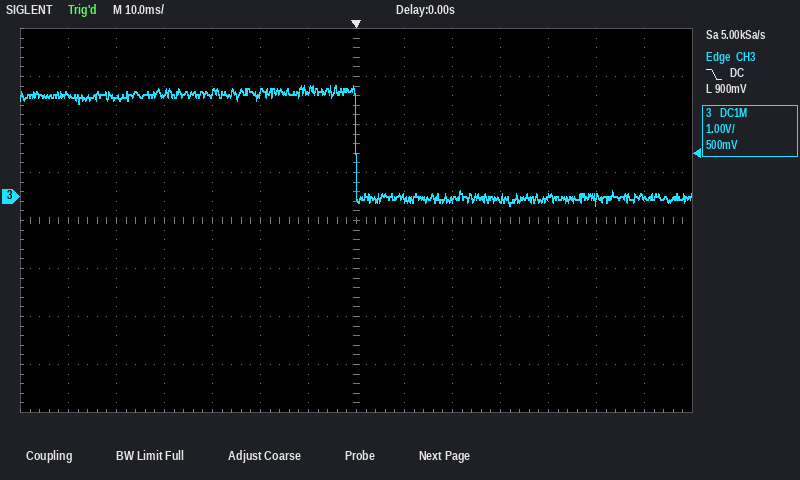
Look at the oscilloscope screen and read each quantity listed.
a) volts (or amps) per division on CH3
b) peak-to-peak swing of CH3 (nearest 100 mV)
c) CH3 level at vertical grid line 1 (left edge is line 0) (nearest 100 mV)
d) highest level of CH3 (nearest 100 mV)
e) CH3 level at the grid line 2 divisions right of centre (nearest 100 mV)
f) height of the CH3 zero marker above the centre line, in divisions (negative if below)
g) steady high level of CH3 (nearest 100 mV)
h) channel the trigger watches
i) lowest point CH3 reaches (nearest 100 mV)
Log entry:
1 V
2.5 V
2.1 V
2.3 V
-100 mV
+0.5 div
2.1 V
CH3
-200 mV
